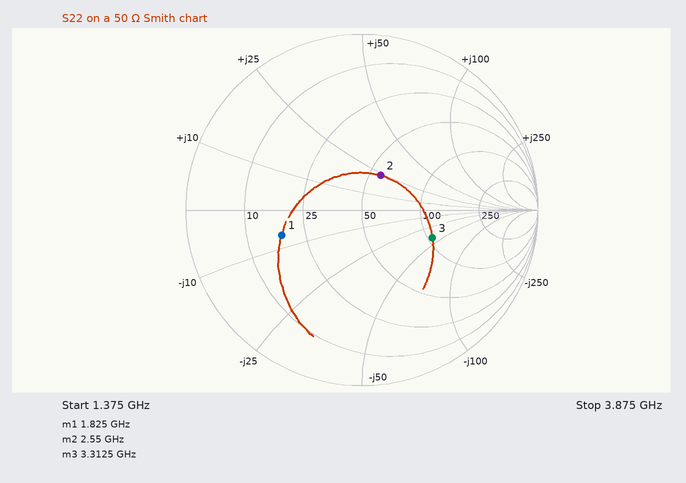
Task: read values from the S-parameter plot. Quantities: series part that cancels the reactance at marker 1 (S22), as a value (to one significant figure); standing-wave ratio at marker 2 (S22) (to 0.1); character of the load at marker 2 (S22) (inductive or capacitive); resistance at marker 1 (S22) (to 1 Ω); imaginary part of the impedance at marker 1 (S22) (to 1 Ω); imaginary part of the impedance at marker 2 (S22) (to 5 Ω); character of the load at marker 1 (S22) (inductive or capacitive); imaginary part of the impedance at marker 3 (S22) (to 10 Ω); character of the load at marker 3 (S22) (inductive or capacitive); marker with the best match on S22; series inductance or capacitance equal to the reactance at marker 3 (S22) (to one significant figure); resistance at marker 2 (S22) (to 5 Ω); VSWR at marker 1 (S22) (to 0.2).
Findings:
600 pH
1.6
inductive
18 Ω
-7 Ω
+25 Ω
capacitive
-40 Ω
capacitive
marker 2
1 pF
55 Ω
2.8
